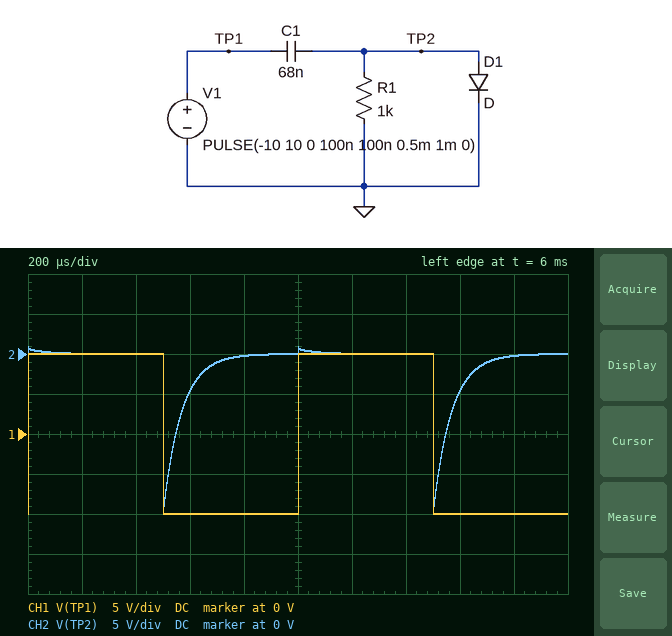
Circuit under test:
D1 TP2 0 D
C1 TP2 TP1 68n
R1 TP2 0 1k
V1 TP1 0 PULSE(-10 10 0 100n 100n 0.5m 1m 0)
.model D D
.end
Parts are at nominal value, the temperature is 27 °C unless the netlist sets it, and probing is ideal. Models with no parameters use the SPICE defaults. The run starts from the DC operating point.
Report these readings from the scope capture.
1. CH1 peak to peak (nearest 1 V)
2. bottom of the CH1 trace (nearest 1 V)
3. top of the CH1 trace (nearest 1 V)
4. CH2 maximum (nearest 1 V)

20 V
-10 V
10 V
1 V
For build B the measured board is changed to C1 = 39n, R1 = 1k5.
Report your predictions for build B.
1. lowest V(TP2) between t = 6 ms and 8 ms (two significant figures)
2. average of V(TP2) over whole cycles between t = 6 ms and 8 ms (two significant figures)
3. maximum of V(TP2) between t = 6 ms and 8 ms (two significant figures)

-20 V
-1.1 V
900 mV
